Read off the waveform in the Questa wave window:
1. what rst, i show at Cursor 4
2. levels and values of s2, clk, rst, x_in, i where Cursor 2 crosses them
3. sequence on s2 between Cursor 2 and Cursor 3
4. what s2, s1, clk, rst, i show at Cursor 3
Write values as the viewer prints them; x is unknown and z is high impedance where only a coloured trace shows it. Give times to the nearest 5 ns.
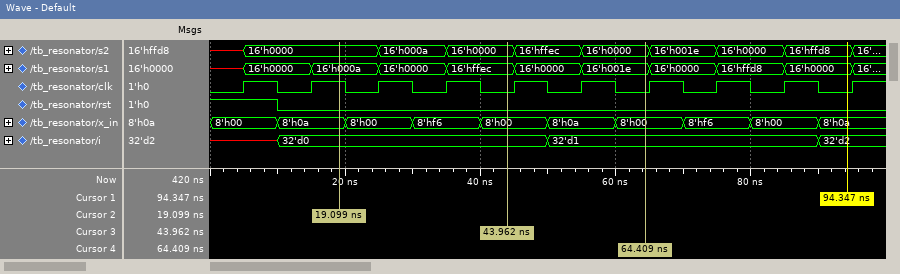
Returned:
rst=0, i=32'd1
s2=16'h0000, clk=1, rst=0, x_in=8'h0a, i=32'd0
16'h0000, 16'h000a, 16'h0000
s2=16'h0000, s1=16'hffec, clk=0, rst=0, i=32'd0
